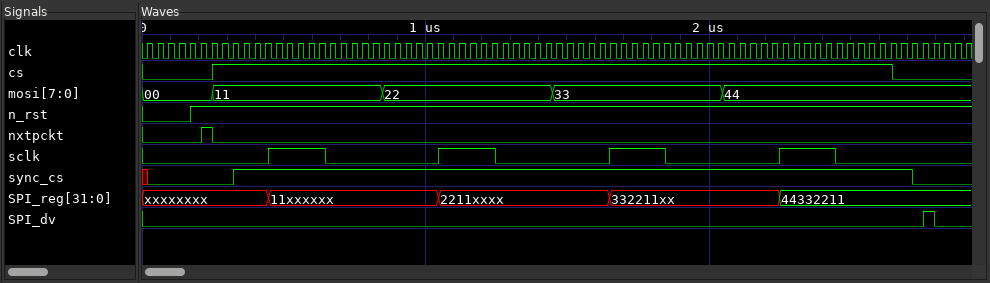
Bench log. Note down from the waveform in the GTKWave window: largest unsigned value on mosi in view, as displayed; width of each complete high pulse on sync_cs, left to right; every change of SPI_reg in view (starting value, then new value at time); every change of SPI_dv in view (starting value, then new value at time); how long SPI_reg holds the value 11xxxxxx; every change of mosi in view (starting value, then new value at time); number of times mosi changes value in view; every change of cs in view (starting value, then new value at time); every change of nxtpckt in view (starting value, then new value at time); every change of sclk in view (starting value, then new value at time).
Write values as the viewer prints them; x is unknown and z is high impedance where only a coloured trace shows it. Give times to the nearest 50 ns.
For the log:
44
2400 ns
xxxxxxxx, 11xxxxxx at 450 ns, 2211xxxx at 1050 ns, 332211xx at 1650 ns, 44332211 at 2250 ns
0, 1 at 2750 ns, 0 at 2800 ns
600 ns
00, 11 at 250 ns, 22 at 850 ns, 33 at 1450 ns, 44 at 2050 ns
4
0, 1 at 250 ns, 0 at 2650 ns
0, 1 at 200 ns, 0 at 250 ns
0, 1 at 450 ns, 0 at 650 ns, 1 at 1050 ns, 0 at 1250 ns, 1 at 1650 ns, 0 at 1850 ns, 1 at 2250 ns, 0 at 2450 ns
